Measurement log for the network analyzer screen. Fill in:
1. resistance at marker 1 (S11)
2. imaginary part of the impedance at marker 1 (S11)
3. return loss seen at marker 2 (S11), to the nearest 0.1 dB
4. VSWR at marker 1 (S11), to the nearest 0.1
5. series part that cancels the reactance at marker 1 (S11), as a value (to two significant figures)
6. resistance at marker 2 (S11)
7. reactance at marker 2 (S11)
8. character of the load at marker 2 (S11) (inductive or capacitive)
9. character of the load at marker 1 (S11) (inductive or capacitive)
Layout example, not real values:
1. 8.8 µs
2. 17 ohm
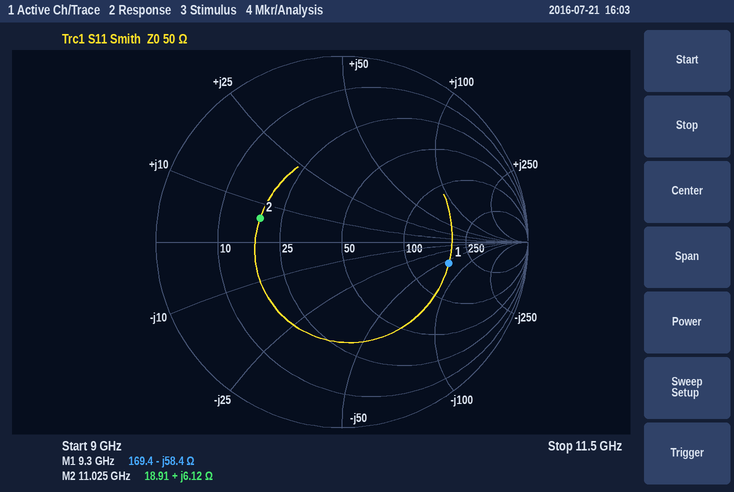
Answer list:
1. 169.4 Ω
2. -58.4 Ω
3. 6.8 dB
4. 3.8
5. 1.00 nH
6. 18.91 Ω
7. +6.12 Ω
8. inductive
9. capacitive
